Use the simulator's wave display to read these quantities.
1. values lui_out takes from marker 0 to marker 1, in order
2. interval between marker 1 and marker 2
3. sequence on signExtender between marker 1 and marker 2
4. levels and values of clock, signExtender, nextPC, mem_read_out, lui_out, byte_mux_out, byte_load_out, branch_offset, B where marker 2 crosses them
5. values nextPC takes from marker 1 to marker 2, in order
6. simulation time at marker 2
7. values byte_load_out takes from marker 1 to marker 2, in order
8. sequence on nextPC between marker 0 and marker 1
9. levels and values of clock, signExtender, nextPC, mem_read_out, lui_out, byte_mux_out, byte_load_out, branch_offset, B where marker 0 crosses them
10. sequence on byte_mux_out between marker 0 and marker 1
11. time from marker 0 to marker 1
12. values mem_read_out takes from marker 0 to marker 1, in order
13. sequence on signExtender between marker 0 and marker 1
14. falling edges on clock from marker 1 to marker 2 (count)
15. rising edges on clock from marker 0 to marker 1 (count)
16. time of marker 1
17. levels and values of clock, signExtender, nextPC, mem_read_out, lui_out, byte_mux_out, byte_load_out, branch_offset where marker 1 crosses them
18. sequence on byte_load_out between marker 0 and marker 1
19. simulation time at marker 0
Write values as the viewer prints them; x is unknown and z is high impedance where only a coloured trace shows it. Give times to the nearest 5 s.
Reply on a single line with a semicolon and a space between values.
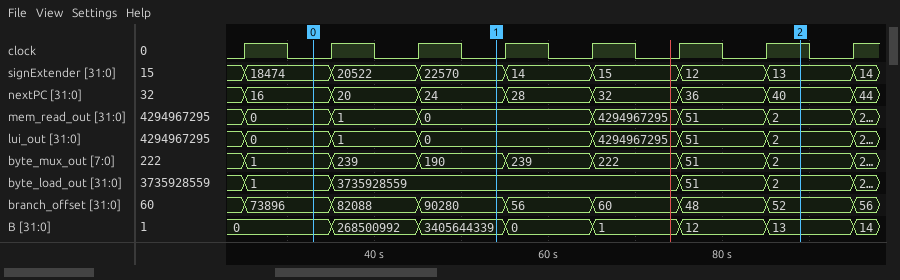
0, 1, 0; 35 s; 22570, 14, 15, 12, 13; clock=1, signExtender=13, nextPC=40, mem_read_out=2, lui_out=2, byte_mux_out=2, byte_load_out=2, branch_offset=52, B=13; 24, 28, 32, 36, 40; 90 s; 3735928559, 51, 2; 16, 20, 24; clock=0, signExtender=18474, nextPC=16, mem_read_out=0, lui_out=0, byte_mux_out=1, byte_load_out=1, branch_offset=73896, B=0; 1, 239, 190; 20 s; 0, 1, 0; 18474, 20522, 22570; 3; 2; 55 s; clock=0, signExtender=22570, nextPC=24, mem_read_out=0, lui_out=0, byte_mux_out=190, byte_load_out=3735928559, branch_offset=90280; 1, 3735928559; 35 s
